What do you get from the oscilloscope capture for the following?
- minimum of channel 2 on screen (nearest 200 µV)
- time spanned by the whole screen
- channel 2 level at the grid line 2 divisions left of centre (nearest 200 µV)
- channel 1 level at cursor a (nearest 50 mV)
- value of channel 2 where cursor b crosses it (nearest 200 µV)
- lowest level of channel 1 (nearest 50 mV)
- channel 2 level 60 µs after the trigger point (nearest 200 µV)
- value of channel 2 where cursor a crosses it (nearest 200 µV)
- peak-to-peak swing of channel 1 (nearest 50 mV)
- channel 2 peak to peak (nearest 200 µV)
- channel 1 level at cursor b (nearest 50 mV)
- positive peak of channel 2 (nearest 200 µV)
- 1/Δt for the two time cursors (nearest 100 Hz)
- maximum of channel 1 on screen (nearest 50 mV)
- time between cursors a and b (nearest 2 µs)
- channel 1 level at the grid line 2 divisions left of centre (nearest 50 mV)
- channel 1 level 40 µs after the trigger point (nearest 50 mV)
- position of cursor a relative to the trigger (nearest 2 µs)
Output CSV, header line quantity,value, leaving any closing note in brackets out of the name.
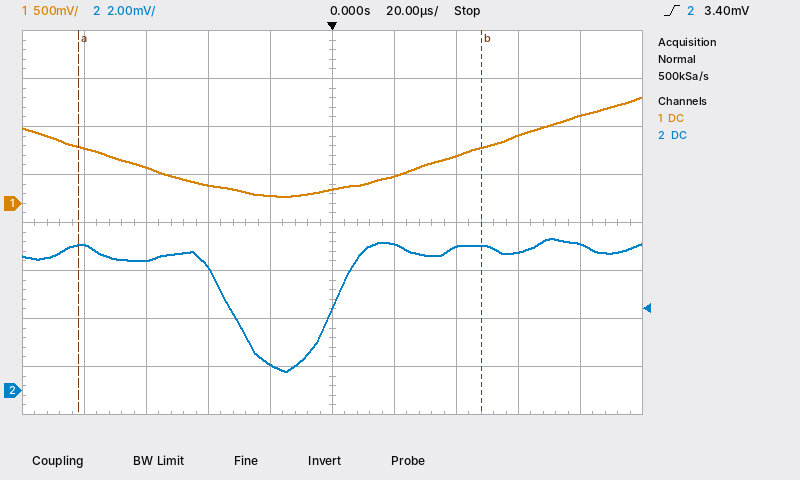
quantity,value
minimum of channel 2 on screen,800 µV
time spanned by the whole screen,200 µs
channel 2 level at the grid line 2 divisions left of centre,5.2 mV
channel 1 level at cursor a,600 mV
value of channel 2 where cursor b crosses it,6.0 mV
lowest level of channel 1,50 mV
channel 2 level 60 µs after the trigger point,5.8 mV
value of channel 2 where cursor a crosses it,6.0 mV
peak-to-peak swing of channel 1,1.05 V
channel 2 peak to peak,5.6 mV
channel 1 level at cursor b,600 mV
positive peak of channel 2,6.4 mV
1/Δt for the two time cursors,7.7 kHz
maximum of channel 1 on screen,1.10 V
time between cursors a and b,130 µs
channel 1 level at the grid line 2 divisions left of centre,200 mV
channel 1 level 40 µs after the trigger point,500 mV
position of cursor a relative to the trigger,-82 µs
